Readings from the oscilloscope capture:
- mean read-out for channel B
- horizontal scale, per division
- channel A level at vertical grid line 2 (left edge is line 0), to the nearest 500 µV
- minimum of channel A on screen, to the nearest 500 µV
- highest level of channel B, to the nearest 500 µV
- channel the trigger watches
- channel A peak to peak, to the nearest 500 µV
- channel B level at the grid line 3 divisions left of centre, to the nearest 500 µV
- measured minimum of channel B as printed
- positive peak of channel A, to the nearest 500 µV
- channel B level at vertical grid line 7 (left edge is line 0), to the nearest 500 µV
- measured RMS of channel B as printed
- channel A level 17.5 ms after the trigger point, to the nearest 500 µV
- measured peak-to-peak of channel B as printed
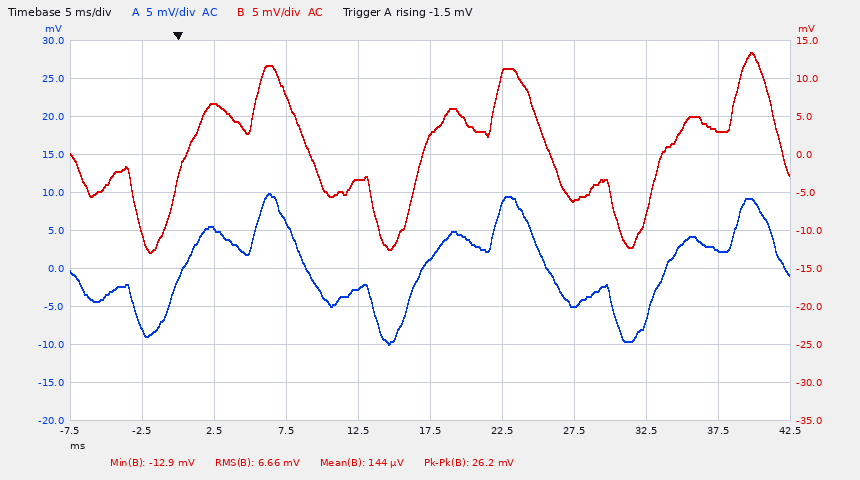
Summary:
144 µV
5 ms
5.0 mV
-10.0 mV
13.5 mV
channel A
20.0 mV
6.5 mV
-12.9 mV
10.0 mV
-6.0 mV
6.66 mV
1.5 mV
26.2 mV
